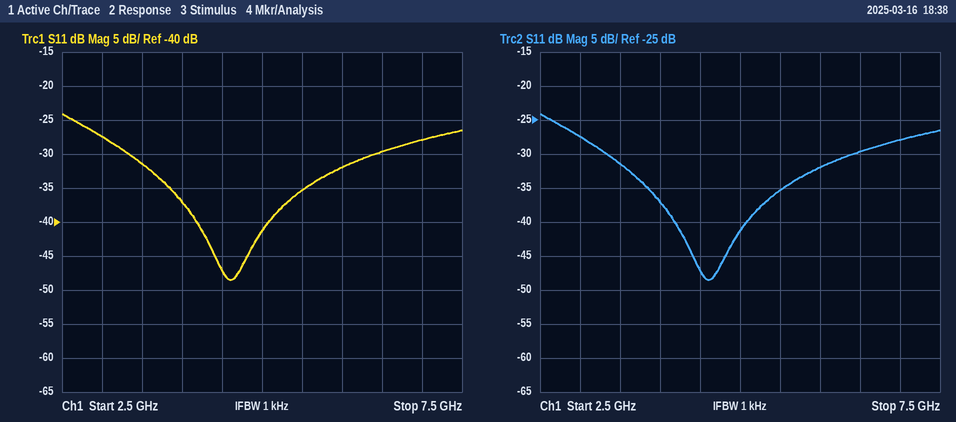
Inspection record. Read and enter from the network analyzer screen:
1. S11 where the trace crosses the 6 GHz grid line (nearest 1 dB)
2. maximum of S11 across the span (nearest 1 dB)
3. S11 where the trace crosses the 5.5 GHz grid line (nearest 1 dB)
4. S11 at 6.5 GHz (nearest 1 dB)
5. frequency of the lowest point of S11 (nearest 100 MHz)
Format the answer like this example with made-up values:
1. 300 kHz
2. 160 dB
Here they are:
1. -32 dB
2. -24 dB
3. -35 dB
4. -30 dB
5. 4.6 GHz
